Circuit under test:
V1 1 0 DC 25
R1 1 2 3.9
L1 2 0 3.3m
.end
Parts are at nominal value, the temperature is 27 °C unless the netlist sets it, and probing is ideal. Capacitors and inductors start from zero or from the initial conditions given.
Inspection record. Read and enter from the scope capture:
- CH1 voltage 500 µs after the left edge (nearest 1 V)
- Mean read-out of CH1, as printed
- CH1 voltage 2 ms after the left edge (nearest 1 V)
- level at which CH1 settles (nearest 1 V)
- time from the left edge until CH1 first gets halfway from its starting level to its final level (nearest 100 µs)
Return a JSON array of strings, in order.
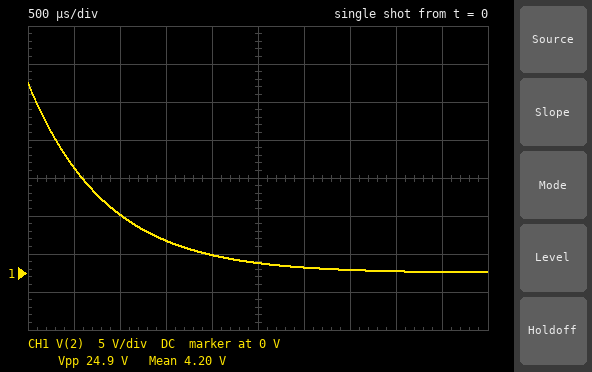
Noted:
["14 V", "4.20 V", "2 V", "0 V", "600 µs"]
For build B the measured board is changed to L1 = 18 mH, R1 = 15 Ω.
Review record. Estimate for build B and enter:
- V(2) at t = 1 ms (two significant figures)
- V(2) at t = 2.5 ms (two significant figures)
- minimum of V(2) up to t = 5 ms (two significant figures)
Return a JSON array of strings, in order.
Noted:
["11 V", "3.1 V", "390 mV"]
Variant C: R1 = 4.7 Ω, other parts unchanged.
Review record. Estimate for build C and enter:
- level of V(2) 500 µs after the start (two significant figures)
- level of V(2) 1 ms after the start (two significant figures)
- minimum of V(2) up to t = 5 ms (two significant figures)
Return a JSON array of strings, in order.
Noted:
["12 V", "6.0 V", "20 mV"]
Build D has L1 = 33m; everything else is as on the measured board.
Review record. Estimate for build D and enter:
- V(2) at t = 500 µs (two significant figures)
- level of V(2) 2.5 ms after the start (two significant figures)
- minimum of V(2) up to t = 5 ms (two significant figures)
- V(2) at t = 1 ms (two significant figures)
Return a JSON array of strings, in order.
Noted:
["24 V", "19 V", "14 V", "22 V"]
